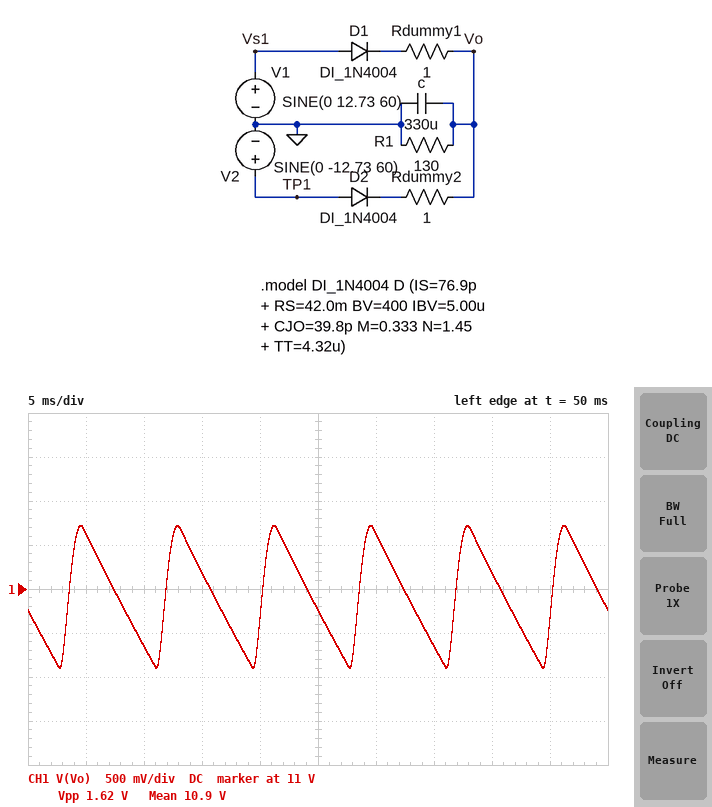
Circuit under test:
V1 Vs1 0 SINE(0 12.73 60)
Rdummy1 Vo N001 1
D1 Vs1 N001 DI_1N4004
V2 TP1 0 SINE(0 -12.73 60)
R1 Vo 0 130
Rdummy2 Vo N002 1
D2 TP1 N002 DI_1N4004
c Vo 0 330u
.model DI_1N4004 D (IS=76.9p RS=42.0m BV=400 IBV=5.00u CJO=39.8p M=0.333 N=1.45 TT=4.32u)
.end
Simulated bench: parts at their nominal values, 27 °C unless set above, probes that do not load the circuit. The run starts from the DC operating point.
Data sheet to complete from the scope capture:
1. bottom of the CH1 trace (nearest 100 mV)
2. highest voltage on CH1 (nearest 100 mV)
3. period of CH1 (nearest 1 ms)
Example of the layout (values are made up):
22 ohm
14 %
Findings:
10.1 V
11.7 V
8 ms
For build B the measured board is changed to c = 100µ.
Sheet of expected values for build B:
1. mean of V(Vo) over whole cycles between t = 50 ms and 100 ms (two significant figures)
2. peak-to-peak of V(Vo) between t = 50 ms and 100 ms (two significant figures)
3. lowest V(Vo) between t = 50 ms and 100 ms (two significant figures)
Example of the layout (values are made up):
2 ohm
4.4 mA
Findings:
9.9 V
4.2 V
7.7 V
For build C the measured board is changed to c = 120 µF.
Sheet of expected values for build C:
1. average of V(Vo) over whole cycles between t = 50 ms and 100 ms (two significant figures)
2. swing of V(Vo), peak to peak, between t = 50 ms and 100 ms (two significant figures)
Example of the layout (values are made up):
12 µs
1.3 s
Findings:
10 V
3.7 V
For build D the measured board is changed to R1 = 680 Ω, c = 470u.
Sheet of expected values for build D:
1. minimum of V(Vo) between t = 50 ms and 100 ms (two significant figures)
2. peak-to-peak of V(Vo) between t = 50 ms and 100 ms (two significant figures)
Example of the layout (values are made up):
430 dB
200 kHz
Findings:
12 V
260 mV
